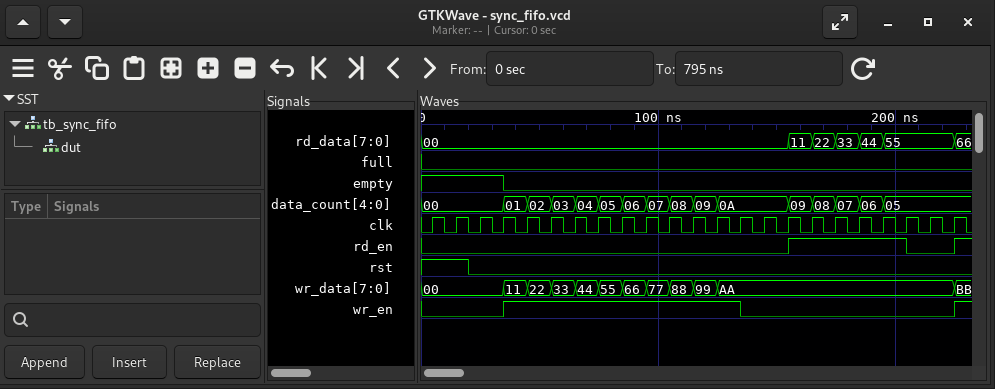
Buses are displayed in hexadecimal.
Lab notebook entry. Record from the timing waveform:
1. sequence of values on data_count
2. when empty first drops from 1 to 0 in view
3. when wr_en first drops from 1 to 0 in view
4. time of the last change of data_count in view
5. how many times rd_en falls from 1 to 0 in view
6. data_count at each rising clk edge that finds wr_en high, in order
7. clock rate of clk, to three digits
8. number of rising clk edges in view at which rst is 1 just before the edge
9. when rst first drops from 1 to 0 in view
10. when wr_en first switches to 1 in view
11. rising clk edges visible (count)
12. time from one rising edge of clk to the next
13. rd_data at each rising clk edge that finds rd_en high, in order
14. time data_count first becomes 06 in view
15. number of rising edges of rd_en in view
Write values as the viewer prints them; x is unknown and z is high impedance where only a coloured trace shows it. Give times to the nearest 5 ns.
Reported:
00, 01, 02, 03, 04, 05, 06, 07, 08, 09, 0A, 09, 08, 07, 06, 05
35 ns
135 ns
195 ns
1
01, 02, 03, 04, 05, 06, 07, 08, 09, 0A
100 MHz
2
20 ns
35 ns
23
10 ns
11, 22, 33, 44, 55
85 ns
2
